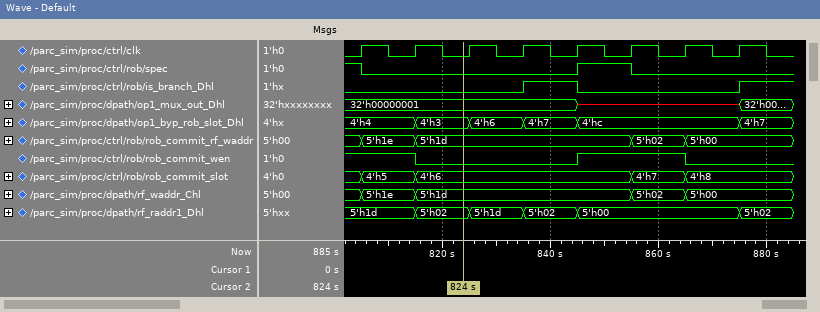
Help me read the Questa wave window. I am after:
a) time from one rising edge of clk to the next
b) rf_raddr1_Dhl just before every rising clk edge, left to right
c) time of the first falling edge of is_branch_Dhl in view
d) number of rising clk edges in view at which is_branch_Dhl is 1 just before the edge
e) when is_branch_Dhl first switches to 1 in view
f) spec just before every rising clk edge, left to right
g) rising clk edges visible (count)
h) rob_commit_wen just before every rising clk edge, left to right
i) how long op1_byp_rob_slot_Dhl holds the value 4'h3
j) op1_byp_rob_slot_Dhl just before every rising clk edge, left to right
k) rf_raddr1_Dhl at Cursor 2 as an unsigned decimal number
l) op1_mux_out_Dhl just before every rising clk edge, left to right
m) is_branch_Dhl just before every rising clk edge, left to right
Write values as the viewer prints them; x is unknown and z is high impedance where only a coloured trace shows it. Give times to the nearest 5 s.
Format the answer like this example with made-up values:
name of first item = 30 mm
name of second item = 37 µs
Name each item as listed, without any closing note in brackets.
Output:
time from one rising edge of clk to the next = 10 s
rf_raddr1_Dhl just before every rising clk edge, left to right = 5'h1d, 5'h1d, 5'h02, 5'h1d, 5'h02, 5'h00, 5'h00, 5'h00
time of the first falling edge of is_branch_Dhl in view = 845 s
number of rising clk edges in view at which is_branch_Dhl is 1 just before the edge = 1
when is_branch_Dhl first switches to 1 in view = 835 s
spec just before every rising clk edge, left to right = 1 0 0 0 0 1 0 0
rising clk edges visible = 8
rob_commit_wen just before every rising clk edge, left to right = 1 1 0 0 0 1 1 0
how long op1_byp_rob_slot_Dhl holds the value 4'h3 = 10 s
op1_byp_rob_slot_Dhl just before every rising clk edge, left to right = 4'h4, 4'h4, 4'h3, 4'h6, 4'h7, 4'hc, 4'hc, 4'hc
rf_raddr1_Dhl at Cursor 2 as an unsigned decimal number = 2
op1_mux_out_Dhl just before every rising clk edge, left to right = 32'h00000001, 32'h00000001, 32'h00000001, 32'h00000001, 32'h00000001, x, x, x
is_branch_Dhl just before every rising clk edge, left to right = 0 0 0 0 1 0 0 0
